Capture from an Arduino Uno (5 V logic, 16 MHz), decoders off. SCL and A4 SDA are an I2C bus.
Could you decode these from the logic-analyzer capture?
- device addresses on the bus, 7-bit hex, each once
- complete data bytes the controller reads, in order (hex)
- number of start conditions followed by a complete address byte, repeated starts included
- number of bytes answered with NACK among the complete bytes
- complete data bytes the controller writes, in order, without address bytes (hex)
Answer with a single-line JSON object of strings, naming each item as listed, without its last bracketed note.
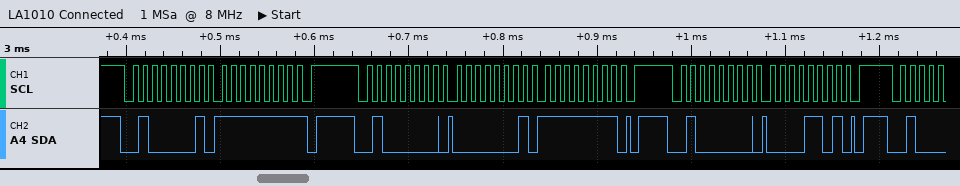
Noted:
{"device addresses on the bus, 7-bit hex, each once": "0x20", "complete data bytes the controller reads, in order": "FF", "number of start conditions followed by a complete address byte, repeated starts included": "3", "number of bytes answered with NACK among the complete bytes": "1", "complete data bytes the controller writes, in order, without address bytes": "01 FF 0D"}
